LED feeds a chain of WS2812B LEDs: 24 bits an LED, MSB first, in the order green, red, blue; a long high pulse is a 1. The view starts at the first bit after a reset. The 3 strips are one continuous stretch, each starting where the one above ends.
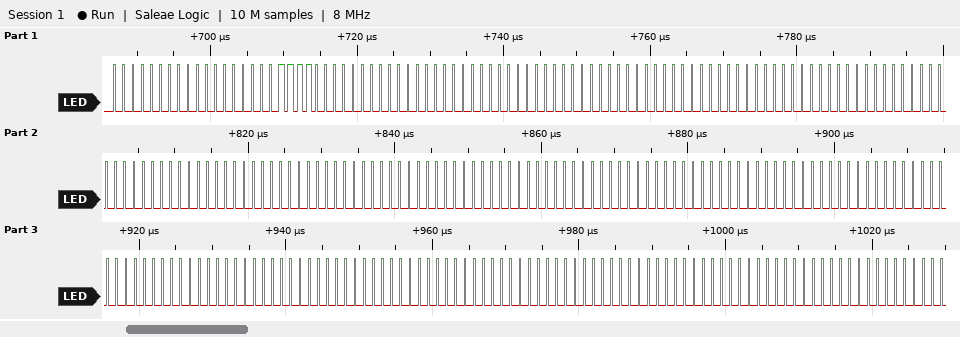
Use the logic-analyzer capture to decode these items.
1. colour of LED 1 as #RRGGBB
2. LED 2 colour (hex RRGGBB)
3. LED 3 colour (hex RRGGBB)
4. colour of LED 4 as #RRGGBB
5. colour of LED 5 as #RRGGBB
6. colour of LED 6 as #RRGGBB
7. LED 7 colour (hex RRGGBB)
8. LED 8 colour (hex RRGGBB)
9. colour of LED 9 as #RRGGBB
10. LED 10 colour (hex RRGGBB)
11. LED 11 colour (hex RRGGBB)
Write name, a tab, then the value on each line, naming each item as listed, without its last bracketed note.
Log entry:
colour of LED 1 as #RRGGBB	#00003C
LED 2 colour	#000000
LED 3 colour	#000000
colour of LED 4 as #RRGGBB	#000000
colour of LED 5 as #RRGGBB	#000000
colour of LED 6 as #RRGGBB	#000000
LED 7 colour	#000000
LED 8 colour	#000000
colour of LED 9 as #RRGGBB	#000000
LED 10 colour	#000000
LED 11 colour	#000000
